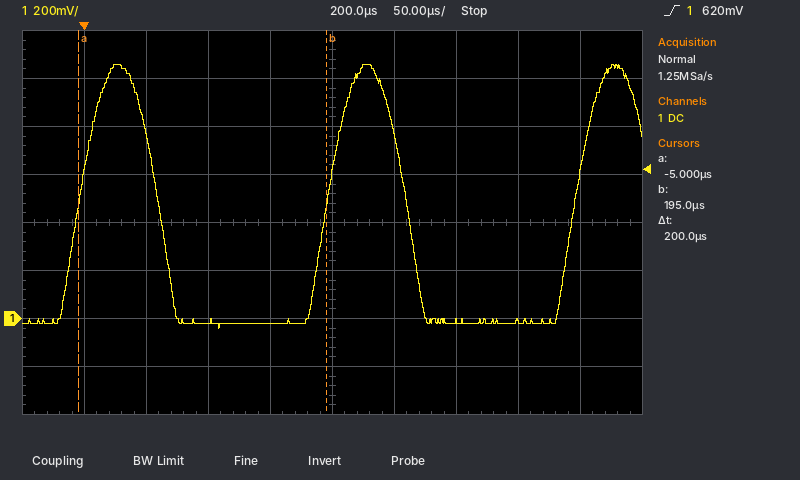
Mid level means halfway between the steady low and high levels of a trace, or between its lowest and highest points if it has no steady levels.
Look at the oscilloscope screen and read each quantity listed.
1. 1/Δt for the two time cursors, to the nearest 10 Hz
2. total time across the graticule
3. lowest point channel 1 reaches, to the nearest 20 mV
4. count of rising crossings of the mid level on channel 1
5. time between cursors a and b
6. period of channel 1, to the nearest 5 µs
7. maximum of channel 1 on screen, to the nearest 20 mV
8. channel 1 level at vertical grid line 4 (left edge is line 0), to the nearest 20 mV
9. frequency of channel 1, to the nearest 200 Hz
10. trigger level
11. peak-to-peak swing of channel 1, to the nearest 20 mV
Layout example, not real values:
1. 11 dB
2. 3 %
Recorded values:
1. 5.00 kHz
2. 500 µs
3. -40 mV
4. 3
5. 200 µs
6. 200 µs
7. 1.06 V
8. -20 mV
9. 5.0 kHz
10. 620 mV
11. 1.10 V
